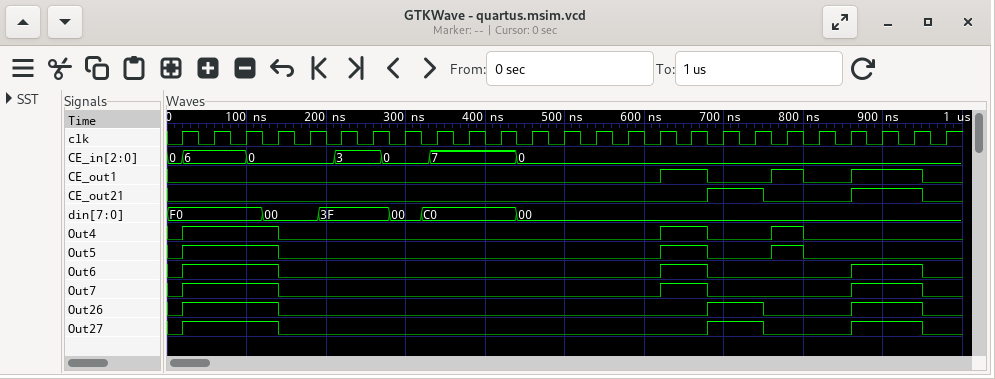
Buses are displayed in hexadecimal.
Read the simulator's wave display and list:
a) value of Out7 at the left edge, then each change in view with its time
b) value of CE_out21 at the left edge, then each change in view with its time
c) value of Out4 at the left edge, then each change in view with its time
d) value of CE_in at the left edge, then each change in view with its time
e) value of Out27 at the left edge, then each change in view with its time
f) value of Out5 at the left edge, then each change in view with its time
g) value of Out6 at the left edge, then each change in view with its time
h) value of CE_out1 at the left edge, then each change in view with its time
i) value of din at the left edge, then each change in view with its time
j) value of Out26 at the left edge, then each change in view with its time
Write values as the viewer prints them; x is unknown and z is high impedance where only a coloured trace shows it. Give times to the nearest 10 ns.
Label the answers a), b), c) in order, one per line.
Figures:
a) 0, 1 at 20 ns, 0 at 140 ns, 1 at 620 ns, 0 at 680 ns, 1 at 860 ns, 0 at 950 ns
b) 0, 1 at 680 ns, 0 at 750 ns, 1 at 860 ns, 0 at 950 ns
c) 0, 1 at 20 ns, 0 at 140 ns, 1 at 620 ns, 0 at 680 ns, 1 at 760 ns, 0 at 800 ns
d) 0, 6 at 20 ns, 0 at 100 ns, 3 at 210 ns, 0 at 270 ns, 7 at 330 ns, 0 at 440 ns
e) 0, 1 at 20 ns, 0 at 140 ns, 1 at 680 ns, 0 at 750 ns, 1 at 860 ns, 0 at 950 ns
f) 0, 1 at 20 ns, 0 at 140 ns, 1 at 620 ns, 0 at 680 ns, 1 at 760 ns, 0 at 800 ns
g) 0, 1 at 20 ns, 0 at 140 ns, 1 at 620 ns, 0 at 680 ns, 1 at 860 ns, 0 at 950 ns
h) 0, 1 at 620 ns, 0 at 680 ns, 1 at 760 ns, 0 at 800 ns, 1 at 860 ns, 0 at 950 ns
i) F0, 00 at 120 ns, 3F at 190 ns, 00 at 280 ns, C0 at 320 ns, 00 at 440 ns
j) 0, 1 at 20 ns, 0 at 140 ns, 1 at 680 ns, 0 at 750 ns, 1 at 860 ns, 0 at 950 ns
